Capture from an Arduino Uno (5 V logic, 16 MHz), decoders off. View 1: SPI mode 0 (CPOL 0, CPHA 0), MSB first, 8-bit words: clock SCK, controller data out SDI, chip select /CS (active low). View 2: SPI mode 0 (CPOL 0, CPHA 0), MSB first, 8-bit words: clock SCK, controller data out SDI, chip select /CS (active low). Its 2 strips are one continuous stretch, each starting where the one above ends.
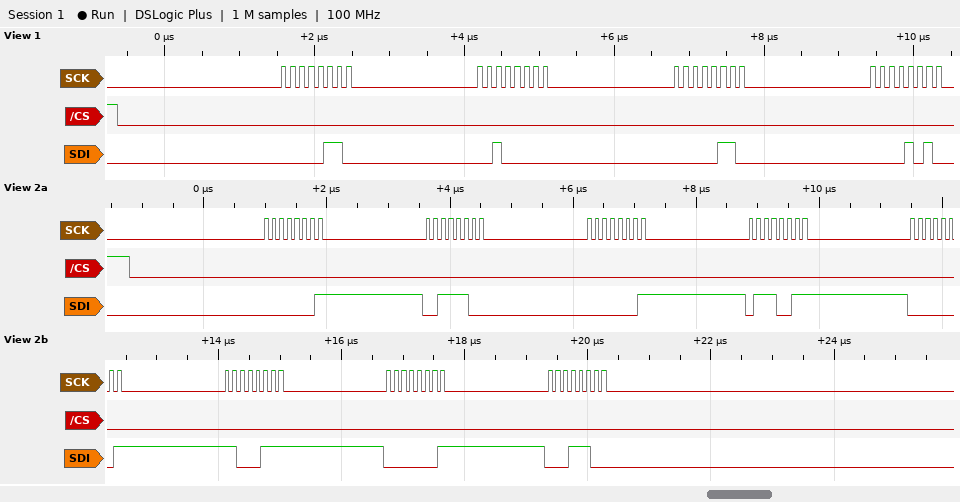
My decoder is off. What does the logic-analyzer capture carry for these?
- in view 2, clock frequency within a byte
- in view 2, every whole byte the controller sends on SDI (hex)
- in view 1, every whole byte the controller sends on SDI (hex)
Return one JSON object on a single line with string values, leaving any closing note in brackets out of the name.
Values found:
{"in view 2, clock frequency within a byte": "8 MHz", "in view 2, every whole byte the controller sends on SDI": "0x01 0x3C 0x01 0x73 0x01 0xC7 0x01 0x1C", "in view 1, every whole byte the controller sends on SDI": "06 20 06 0A"}
